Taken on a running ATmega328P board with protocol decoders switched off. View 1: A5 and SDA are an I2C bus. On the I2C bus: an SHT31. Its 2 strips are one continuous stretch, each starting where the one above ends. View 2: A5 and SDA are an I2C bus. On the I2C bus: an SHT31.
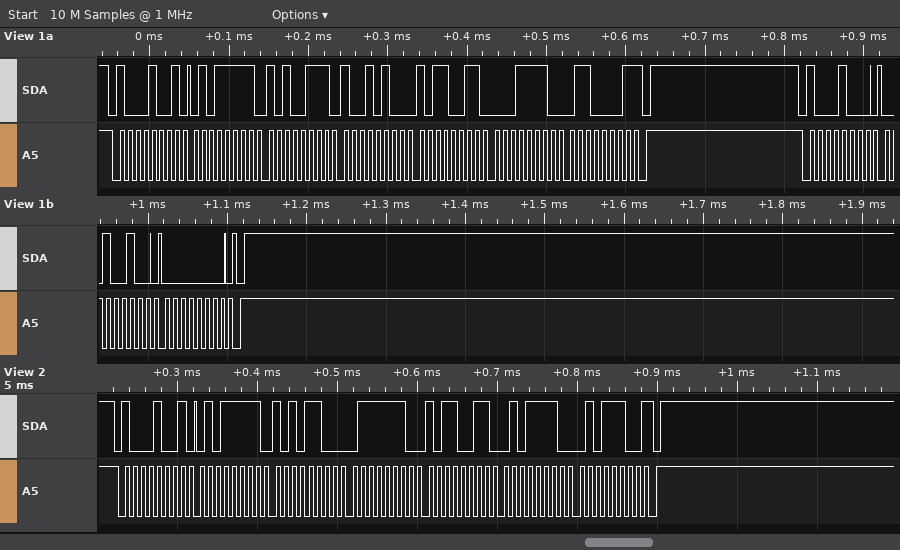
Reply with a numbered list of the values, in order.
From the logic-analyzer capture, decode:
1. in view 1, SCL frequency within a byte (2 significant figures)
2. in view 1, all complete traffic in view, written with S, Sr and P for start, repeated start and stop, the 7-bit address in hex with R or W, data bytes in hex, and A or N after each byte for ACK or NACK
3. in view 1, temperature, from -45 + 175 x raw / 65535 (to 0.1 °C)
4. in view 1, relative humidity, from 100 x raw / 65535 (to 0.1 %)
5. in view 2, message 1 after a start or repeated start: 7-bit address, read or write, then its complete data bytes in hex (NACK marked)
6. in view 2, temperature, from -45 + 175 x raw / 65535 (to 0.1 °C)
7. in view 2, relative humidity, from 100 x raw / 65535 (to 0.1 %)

1. 100 kHz
2. S 44R A 5F A A7 A 94 A B3 A 1E A 61 N P S 44W A 24 A 00 A P
3. 20.4 °C
4. 70.0 %
5. 0x44 read: 5F AC 7E B3 5E 5C NACK
6. 20.4 °C
7. 70.1 %
